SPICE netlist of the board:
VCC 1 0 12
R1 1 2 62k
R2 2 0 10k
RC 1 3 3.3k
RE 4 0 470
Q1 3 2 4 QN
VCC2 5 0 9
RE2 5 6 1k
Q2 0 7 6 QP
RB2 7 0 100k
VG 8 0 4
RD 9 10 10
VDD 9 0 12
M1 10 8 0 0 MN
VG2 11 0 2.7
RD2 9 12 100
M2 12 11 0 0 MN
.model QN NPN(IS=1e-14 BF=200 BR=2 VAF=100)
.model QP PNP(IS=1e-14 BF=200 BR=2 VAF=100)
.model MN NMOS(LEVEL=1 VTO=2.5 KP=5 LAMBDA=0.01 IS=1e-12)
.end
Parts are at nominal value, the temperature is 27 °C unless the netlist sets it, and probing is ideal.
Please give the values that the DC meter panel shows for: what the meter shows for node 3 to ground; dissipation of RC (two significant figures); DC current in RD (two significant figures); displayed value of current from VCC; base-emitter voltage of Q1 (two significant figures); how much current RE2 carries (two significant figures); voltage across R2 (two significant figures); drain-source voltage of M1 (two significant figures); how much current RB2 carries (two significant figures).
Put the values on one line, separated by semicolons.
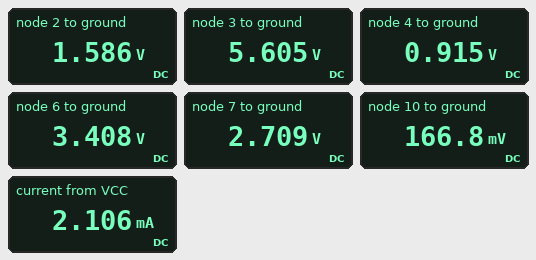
5.605 V; 12 mW; 1.2 A; 2.106 mA; 670 mV; 5.6 mA; 1.6 V; 170 mV; 27 µA
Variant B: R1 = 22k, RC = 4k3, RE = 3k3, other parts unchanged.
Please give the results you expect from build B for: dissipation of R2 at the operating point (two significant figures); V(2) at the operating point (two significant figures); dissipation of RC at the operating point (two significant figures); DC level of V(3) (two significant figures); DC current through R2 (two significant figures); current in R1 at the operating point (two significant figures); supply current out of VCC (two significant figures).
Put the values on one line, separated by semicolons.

1.4 mW; 3.7 V; 3.7 mW; 8.0 V; 370 µA; 380 µA; 1.3 mA
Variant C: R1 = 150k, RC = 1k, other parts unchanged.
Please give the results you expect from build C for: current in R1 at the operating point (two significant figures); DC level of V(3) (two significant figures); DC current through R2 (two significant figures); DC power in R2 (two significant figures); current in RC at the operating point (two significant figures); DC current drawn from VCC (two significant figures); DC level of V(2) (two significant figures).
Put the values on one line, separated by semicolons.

75 µA; 12 V; 74 µA; 55 µW; 260 µA; 330 µA; 740 mV
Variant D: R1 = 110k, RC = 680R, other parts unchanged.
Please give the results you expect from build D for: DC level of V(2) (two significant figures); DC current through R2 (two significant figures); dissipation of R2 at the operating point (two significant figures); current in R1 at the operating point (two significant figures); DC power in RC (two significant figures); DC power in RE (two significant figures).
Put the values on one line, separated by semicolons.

970 mV; 97 µA; 94 µW; 100 µA; 330 µW; 230 µW
